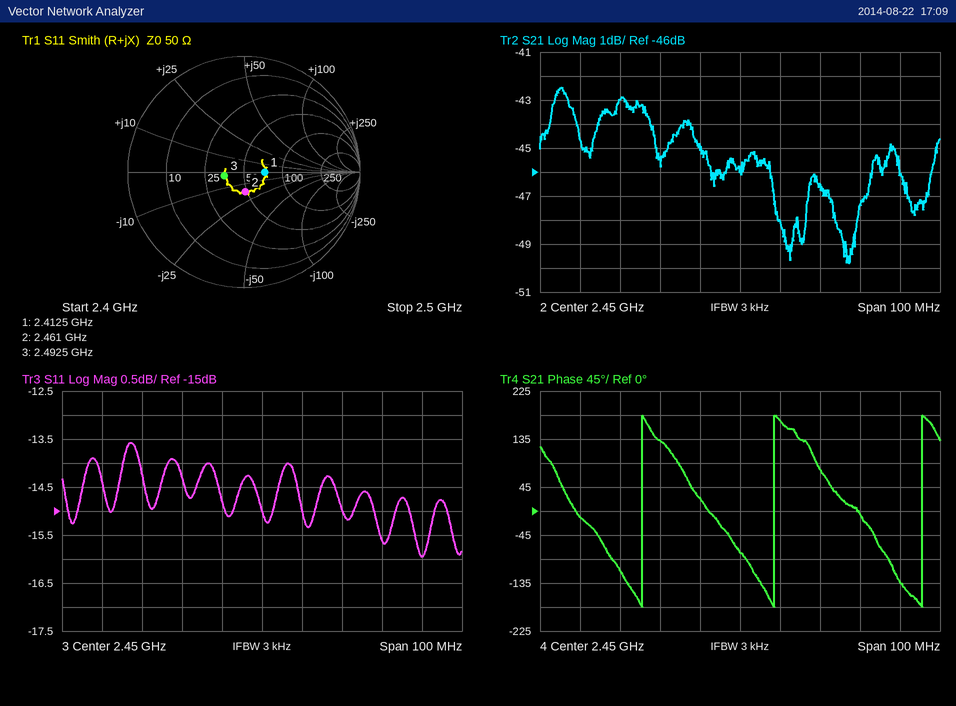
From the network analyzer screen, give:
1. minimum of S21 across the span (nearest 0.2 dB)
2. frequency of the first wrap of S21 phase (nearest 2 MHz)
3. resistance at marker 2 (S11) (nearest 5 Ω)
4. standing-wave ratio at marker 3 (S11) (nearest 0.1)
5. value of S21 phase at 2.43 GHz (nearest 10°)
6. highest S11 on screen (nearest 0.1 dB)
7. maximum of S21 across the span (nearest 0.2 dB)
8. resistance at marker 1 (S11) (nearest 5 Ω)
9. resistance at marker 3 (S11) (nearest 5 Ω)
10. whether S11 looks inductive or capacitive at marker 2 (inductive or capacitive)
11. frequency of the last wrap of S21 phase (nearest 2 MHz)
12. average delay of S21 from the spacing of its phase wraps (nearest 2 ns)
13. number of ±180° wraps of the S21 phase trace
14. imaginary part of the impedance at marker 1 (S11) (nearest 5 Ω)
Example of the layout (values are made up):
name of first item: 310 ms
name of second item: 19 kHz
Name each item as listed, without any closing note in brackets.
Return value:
minimum of S21 across the span: -49.8 dB
frequency of the first wrap of S21 phase: 2.426 GHz
resistance at marker 2 (S11): 50 Ω
standing-wave ratio at marker 3 (S11): 1.4
value of S21 phase at 2.43 GHz: 130°
highest S11 on screen: -13.6 dB
maximum of S21 across the span: -42.4 dB
resistance at marker 1 (S11): 70 Ω
resistance at marker 3 (S11): 35 Ω
whether S11 looks inductive or capacitive at marker 2: capacitive
frequency of the last wrap of S21 phase: 2.496 GHz
average delay of S21 from the spacing of its phase wraps: 28 ns
number of ±180° wraps of the S21 phase trace: 3
imaginary part of the impedance at marker 1 (S11): 0 Ω
